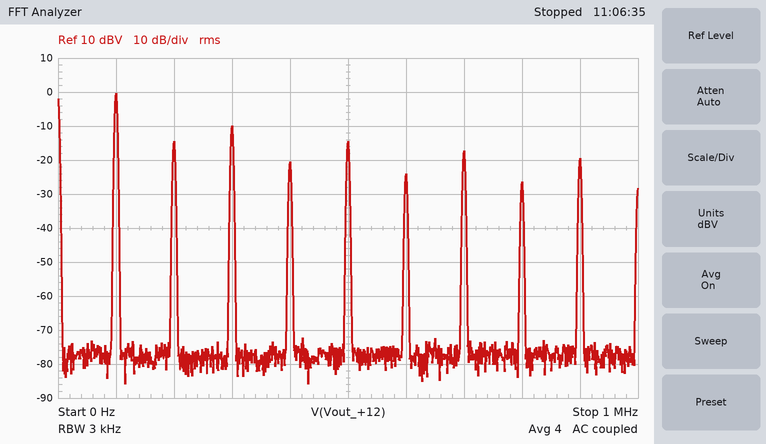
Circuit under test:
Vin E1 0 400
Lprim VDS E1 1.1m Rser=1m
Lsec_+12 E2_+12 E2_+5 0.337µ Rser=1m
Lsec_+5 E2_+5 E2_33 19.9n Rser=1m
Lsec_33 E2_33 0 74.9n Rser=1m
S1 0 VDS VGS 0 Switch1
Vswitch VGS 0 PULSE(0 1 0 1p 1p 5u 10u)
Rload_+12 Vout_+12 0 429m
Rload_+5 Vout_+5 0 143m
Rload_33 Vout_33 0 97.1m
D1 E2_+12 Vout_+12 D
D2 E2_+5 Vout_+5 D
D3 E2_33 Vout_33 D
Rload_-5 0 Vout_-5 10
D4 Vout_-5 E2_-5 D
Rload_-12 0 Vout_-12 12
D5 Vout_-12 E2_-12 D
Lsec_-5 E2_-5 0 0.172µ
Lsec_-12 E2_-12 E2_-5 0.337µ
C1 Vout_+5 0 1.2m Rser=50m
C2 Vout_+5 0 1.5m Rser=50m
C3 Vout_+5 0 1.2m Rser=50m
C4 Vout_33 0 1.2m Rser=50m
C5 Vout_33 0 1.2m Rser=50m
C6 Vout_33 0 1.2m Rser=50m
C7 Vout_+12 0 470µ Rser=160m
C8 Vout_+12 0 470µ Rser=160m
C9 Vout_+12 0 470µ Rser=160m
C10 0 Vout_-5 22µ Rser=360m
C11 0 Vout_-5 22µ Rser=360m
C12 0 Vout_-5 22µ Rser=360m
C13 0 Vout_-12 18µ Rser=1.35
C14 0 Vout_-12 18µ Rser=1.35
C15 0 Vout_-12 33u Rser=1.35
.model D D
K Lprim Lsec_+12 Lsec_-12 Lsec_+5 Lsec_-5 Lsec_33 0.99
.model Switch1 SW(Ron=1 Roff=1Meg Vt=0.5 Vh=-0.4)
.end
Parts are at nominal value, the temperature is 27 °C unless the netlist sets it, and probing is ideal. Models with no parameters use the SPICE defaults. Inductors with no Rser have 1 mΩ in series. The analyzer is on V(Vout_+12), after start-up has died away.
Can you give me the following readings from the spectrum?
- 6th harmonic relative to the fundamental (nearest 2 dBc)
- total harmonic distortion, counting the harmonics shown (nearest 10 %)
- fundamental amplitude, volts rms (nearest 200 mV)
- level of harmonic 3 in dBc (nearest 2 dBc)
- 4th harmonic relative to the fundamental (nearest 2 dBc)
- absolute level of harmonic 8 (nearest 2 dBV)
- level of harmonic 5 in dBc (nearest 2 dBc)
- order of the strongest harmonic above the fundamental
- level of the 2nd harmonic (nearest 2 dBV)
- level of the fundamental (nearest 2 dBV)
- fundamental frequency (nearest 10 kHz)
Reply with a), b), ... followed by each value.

a) -24 dBc
b) 50 %
c) 1.0 V
d) -10 dBc
e) -20 dBc
f) -26 dBV
g) -14 dBc
h) 3
i) -14 dBV
j) 0 dBV
k) 100 kHz
